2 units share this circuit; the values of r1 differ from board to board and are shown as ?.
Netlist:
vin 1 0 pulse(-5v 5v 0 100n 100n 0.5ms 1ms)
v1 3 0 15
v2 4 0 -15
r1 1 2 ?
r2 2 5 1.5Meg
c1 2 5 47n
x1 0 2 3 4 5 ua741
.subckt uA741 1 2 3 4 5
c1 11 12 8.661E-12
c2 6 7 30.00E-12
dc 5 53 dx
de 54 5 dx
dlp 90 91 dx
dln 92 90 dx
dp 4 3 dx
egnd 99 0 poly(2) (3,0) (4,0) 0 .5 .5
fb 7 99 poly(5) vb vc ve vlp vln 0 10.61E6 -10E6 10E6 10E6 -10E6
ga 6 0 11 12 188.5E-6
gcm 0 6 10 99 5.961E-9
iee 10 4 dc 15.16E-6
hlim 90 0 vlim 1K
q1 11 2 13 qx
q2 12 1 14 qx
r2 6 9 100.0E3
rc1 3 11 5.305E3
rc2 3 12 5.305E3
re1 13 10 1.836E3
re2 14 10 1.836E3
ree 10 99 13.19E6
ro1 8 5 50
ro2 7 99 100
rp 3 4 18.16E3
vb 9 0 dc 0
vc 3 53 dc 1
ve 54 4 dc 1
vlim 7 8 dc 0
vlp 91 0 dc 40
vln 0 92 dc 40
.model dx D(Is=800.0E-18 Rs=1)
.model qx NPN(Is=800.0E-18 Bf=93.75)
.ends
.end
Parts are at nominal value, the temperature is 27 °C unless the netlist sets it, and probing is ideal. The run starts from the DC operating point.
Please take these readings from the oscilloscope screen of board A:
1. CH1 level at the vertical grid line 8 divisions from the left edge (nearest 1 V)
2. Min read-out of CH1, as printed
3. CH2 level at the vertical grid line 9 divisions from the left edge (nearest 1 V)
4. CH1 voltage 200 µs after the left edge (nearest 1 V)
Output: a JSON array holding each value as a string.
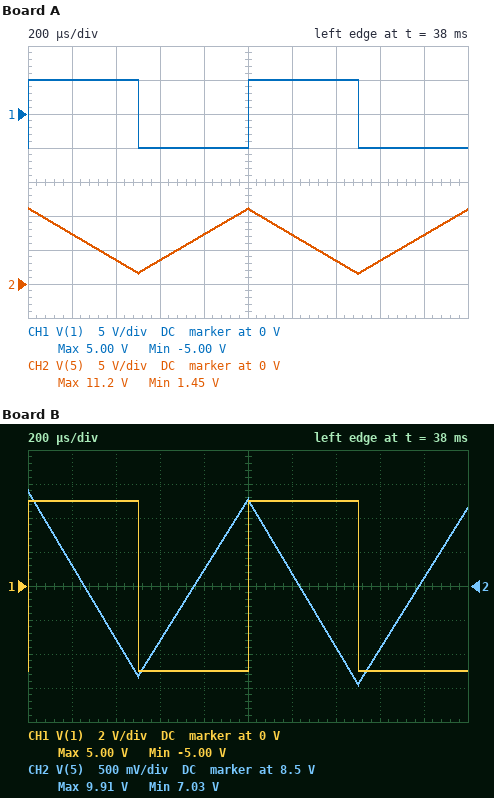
["-5 V", "-5.00 V", "7 V", "5 V"]
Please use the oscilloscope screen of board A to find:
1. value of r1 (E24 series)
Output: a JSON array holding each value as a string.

["5.6 kΩ"]
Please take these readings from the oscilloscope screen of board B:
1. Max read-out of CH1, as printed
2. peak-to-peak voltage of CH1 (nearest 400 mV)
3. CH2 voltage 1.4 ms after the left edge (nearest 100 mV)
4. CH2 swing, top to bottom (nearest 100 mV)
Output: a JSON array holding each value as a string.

["5.00 V", "10.0 V", "7.6 V", "2.9 V"]
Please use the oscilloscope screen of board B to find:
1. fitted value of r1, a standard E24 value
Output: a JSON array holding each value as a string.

["20 kΩ"]
